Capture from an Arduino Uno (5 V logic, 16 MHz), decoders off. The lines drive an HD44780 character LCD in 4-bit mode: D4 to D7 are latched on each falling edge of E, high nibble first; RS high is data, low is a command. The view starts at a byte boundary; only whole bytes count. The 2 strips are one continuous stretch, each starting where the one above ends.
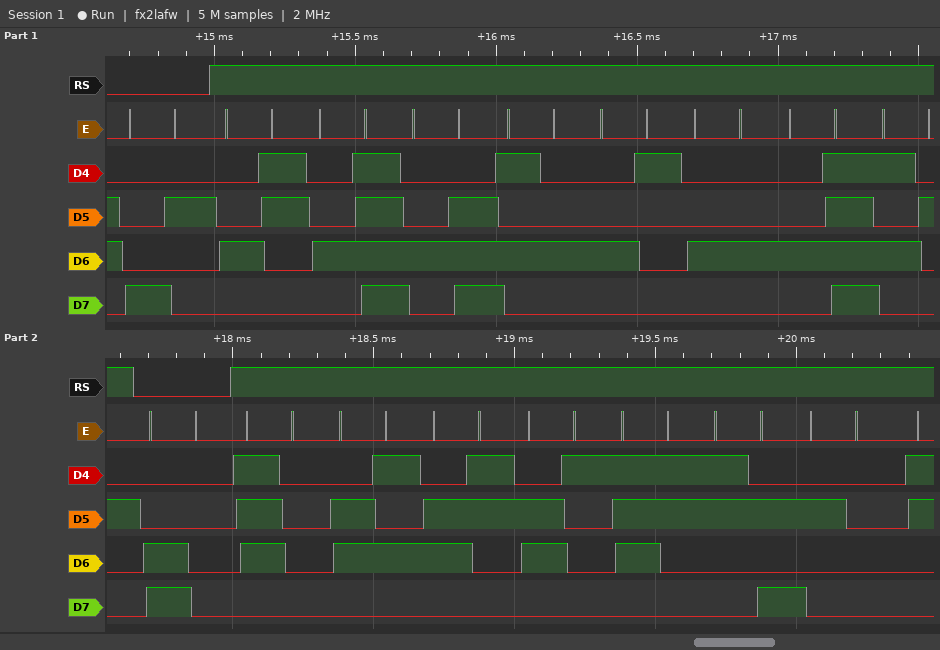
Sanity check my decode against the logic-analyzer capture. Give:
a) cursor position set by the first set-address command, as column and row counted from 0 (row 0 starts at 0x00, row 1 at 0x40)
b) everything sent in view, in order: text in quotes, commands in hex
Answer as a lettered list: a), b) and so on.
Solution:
a) column 2, row 0
b) 0x82 "CONTADOR" 0xC0 "pecas: "
